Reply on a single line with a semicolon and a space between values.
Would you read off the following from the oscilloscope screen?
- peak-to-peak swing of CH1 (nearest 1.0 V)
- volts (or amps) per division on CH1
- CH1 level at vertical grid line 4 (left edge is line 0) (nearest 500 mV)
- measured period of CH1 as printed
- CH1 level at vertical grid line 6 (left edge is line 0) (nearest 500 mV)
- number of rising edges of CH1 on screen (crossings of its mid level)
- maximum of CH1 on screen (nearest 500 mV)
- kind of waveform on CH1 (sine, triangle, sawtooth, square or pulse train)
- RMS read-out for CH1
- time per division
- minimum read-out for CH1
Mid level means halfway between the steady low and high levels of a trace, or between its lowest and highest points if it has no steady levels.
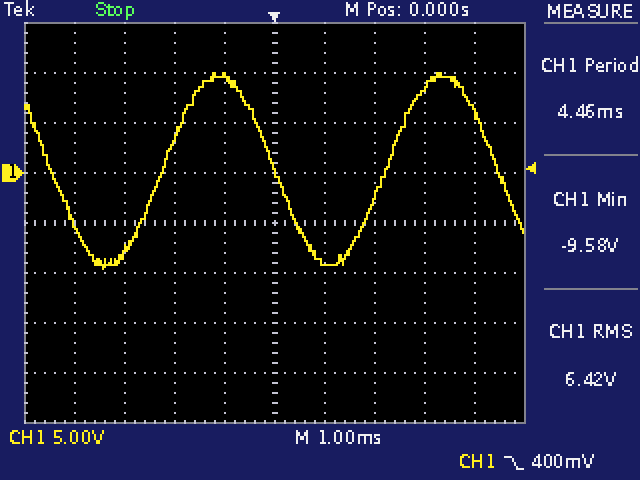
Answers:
20.0 V; 5 V; 9.5 V; 4.46 ms; -9.0 V; 2; 10.0 V; sine; 6.42 V; 1 ms; -9.58 V
